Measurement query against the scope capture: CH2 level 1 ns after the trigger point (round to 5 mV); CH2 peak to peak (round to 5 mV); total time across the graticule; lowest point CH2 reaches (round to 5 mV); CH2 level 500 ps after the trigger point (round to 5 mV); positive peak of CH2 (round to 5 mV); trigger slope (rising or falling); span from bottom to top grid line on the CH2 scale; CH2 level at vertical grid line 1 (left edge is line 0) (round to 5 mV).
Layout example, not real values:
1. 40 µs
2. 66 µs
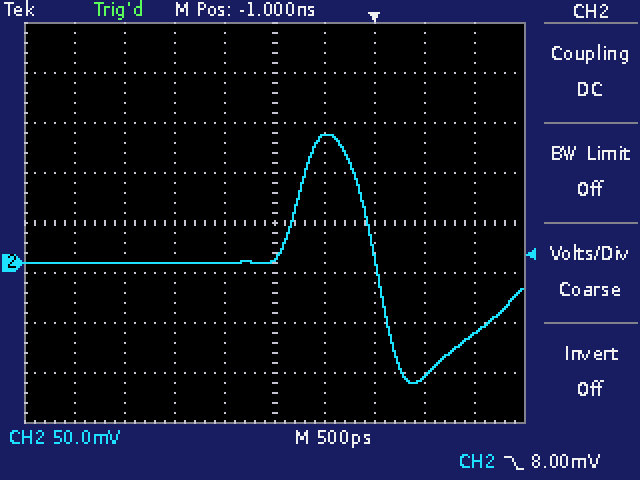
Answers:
1. -70 mV
2. 250 mV
3. 5 ns
4. -120 mV
5. -115 mV
6. 130 mV
7. falling
8. 400 mV
9. 0 mV
